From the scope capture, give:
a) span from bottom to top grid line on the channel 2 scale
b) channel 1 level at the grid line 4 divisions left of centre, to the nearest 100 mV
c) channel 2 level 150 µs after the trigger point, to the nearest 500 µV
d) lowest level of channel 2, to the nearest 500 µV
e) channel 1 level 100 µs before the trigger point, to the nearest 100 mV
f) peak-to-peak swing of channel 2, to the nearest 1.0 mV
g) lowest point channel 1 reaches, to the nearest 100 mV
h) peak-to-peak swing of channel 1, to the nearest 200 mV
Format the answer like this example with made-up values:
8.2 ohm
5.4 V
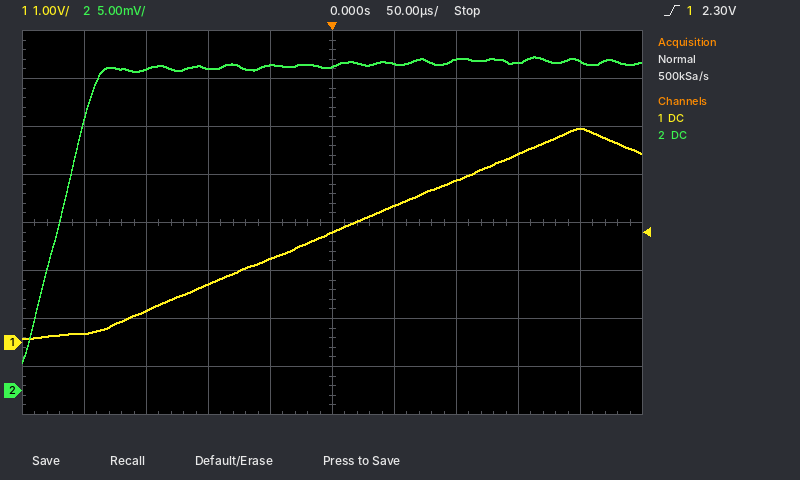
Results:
40 mV
200 mV
34.0 mV
3.0 mV
1.2 V
32.0 mV
100 mV
4.4 V
